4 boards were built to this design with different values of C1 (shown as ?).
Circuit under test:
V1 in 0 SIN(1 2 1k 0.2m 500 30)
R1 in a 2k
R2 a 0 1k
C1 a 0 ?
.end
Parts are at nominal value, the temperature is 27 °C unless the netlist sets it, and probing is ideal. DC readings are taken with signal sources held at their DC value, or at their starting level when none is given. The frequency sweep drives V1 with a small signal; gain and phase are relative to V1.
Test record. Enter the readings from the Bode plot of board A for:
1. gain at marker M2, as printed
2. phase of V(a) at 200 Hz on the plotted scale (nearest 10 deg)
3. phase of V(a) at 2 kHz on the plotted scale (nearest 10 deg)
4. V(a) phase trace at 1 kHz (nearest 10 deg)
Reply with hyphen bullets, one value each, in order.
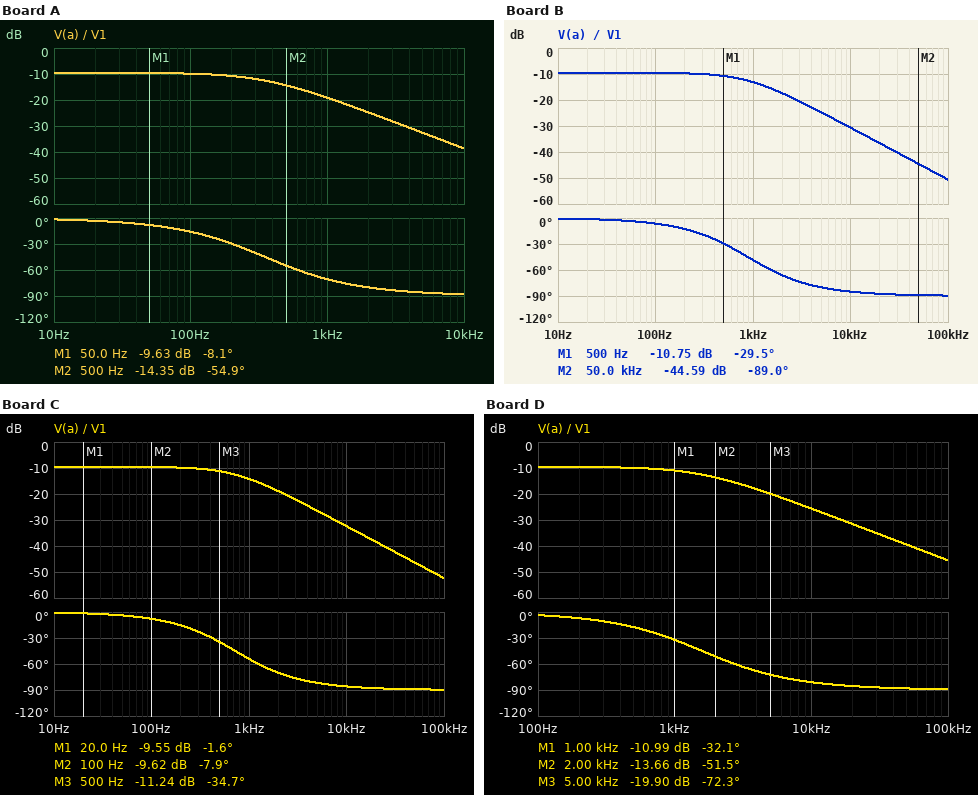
- -14.35 dB
- -30 deg
- -80 deg
- -70 deg
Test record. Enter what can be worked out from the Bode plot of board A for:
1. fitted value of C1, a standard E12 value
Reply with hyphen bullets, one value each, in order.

- 680 nF
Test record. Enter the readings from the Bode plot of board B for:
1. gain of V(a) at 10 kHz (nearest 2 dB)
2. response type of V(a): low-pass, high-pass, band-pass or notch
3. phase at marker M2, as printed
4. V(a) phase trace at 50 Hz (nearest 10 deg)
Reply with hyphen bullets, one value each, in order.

- -30 dB
- low-pass
- -89.0 deg
- 0 deg
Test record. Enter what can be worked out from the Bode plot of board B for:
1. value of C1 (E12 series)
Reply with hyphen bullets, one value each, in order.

- 270 nF
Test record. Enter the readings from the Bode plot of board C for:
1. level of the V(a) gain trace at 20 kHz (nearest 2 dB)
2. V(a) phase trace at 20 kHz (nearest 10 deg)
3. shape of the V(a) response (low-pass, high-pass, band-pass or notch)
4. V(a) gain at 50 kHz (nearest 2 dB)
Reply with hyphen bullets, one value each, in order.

- -38 dB
- -90 deg
- low-pass
- -46 dB
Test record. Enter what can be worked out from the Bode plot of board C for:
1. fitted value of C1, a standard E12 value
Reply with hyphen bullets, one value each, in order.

- 330 nF
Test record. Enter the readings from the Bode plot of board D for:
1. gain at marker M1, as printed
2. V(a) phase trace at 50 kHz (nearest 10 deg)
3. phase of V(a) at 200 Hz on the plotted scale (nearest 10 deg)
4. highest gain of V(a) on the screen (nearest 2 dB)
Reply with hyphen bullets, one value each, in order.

- -10.99 dB
- -90 deg
- -10 deg
- -10 dB
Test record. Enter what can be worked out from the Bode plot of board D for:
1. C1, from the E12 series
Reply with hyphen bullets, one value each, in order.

- 150 nF
